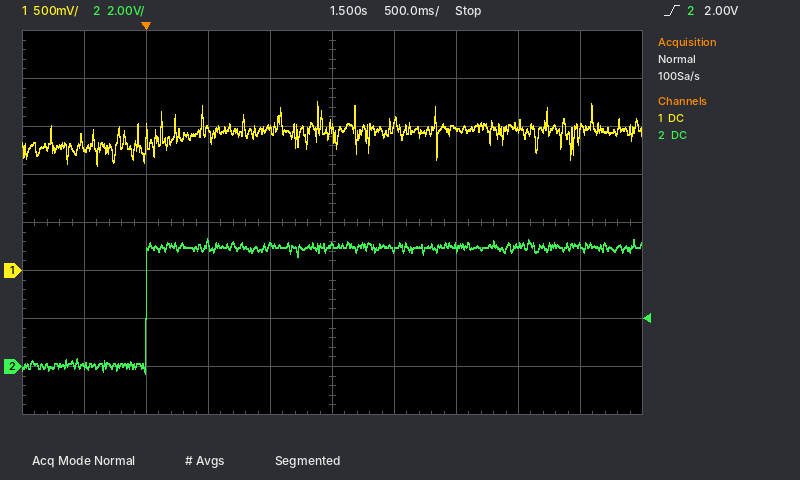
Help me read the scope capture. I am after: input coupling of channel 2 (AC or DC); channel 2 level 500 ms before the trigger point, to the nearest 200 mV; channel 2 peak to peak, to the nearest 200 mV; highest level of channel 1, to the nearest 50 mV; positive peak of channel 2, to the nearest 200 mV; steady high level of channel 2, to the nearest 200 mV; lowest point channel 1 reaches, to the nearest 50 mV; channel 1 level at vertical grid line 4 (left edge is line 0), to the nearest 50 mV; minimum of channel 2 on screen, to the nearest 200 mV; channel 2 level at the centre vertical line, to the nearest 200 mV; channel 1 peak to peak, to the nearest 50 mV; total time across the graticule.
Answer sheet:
DC
0.0 V
5.6 V
1.75 V
5.4 V
5.0 V
1.10 V
1.45 V
-200 mV
5.0 V
650 mV
5 s
